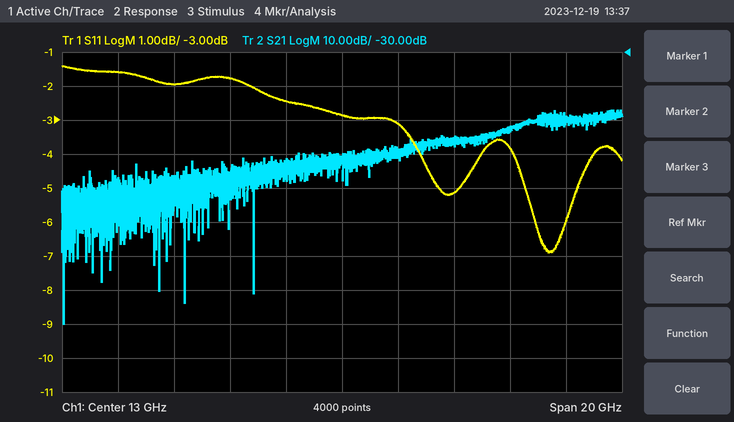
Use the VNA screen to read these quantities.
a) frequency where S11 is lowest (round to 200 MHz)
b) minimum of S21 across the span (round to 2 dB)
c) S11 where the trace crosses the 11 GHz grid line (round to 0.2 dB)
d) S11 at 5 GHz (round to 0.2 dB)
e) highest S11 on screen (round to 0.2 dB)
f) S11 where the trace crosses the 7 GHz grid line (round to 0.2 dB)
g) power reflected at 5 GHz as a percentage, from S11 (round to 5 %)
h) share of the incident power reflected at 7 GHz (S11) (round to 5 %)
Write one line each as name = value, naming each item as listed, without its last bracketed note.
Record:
frequency where S11 is lowest = 20.4 GHz
minimum of S21 across the span = -110 dB
S11 where the trace crosses the 11 GHz grid line = -2.4 dB
S11 at 5 GHz = -1.6 dB
highest S11 on screen = -1.4 dB
S11 where the trace crosses the 7 GHz grid line = -2.0 dB
power reflected at 5 GHz as a percentage, from S11 = 70 %
share of the incident power reflected at 7 GHz (S11) = 65 %
